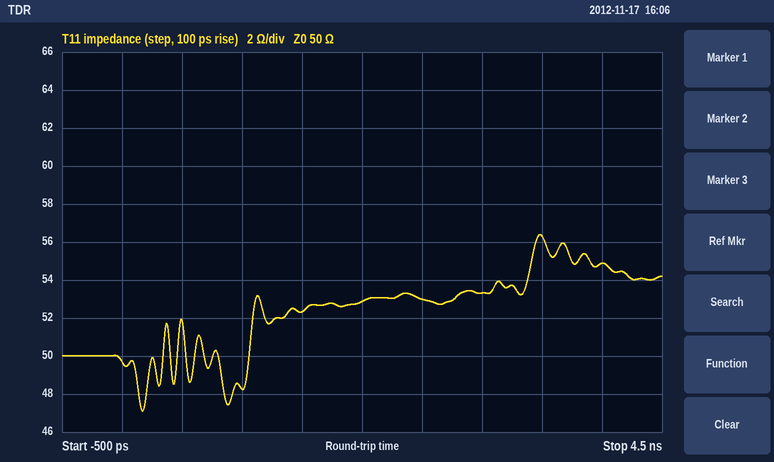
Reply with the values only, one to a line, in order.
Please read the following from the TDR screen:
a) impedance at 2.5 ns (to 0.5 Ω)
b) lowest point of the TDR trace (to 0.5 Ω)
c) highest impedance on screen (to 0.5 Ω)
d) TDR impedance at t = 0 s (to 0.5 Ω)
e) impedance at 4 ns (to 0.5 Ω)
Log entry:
53.0 Ω
47.0 Ω
56.5 Ω
49.5 Ω
55.0 Ω
